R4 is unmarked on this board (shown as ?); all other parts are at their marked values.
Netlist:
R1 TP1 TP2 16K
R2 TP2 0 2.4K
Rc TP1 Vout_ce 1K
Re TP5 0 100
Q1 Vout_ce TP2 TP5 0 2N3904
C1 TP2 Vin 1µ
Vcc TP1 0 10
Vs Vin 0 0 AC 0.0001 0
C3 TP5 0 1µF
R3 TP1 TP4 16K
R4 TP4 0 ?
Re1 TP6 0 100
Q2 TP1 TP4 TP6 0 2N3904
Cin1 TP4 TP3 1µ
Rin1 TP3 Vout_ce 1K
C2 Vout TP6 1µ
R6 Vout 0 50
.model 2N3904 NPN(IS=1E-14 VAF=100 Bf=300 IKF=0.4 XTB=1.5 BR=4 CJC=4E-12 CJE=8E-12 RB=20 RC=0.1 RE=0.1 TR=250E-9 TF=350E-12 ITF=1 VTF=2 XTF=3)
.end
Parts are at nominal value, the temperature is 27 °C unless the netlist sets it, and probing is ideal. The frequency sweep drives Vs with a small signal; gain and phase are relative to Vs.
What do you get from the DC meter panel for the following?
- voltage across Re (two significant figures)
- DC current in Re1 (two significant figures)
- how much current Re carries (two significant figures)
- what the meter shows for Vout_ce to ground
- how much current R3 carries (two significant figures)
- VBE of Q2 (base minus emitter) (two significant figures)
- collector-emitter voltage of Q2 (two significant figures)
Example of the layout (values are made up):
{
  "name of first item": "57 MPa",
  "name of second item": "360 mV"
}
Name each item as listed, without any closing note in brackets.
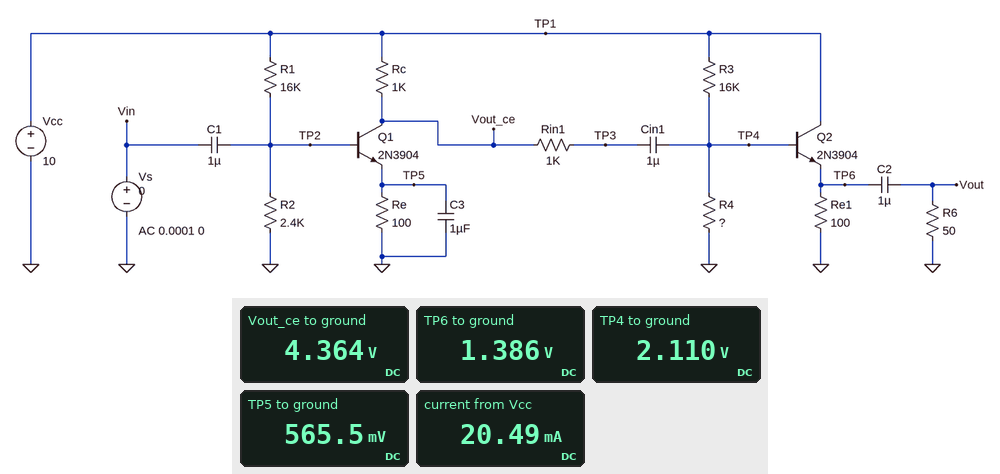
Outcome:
{
  "voltage across Re": "570 mV",
  "DC current in Re1": "14 mA",
  "how much current Re carries": "5.7 mA",
  "what the meter shows for Vout_ce to ground": "4.364 V",
  "how much current R3 carries": "490 µA",
  "VBE of Q2 (base minus emitter)": "720 mV",
  "collector-emitter voltage of Q2": "8.6 V"
}
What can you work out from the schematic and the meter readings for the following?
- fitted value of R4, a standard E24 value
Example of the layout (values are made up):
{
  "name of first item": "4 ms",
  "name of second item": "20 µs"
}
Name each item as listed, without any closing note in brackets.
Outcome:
{
  "fitted value of R4, a standard E24 value": "4.7 kΩ"
}
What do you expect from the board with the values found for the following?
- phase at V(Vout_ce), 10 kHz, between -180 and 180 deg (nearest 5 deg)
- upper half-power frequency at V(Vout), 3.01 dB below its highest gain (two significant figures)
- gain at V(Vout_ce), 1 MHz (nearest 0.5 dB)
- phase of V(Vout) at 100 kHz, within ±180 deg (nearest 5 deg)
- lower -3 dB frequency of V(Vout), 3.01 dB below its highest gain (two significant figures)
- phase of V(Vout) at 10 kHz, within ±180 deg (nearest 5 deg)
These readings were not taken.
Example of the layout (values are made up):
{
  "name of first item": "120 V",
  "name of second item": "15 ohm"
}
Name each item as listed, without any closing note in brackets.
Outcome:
{
  "phase at V(Vout_ce), 10 kHz, between -180 and 180 deg": "-115 deg",
  "upper half-power frequency at V(Vout), 3.01 dB below its highest gain": "7.7 MHz",
  "gain at V(Vout_ce), 1 MHz": "44.0 dB",
  "phase of V(Vout) at 100 kHz, within ±180 deg": "-160 deg",
  "lower -3 dB frequency of V(Vout), 3.01 dB below its highest gain": "33 kHz",
  "phase of V(Vout) at 10 kHz, within ±180 deg": "-100 deg"
}
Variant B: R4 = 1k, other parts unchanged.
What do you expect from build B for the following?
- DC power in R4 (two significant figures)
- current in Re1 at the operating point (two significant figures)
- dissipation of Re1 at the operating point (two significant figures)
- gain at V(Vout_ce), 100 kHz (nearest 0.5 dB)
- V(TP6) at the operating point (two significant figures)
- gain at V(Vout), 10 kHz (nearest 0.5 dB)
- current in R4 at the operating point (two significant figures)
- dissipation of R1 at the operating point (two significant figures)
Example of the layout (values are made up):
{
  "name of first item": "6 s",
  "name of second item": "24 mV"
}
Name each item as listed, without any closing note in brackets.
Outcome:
{
  "DC power in R4": "350 µW",
  "current in Re1 at the operating point": "64 µA",
  "dissipation of Re1 at the operating point": "410 nW",
  "gain at V(Vout_ce), 100 kHz": "42.0 dB",
  "V(TP6) at the operating point": "6.4 mV",
  "gain at V(Vout), 10 kHz": "3.0 dB",
  "current in R4 at the operating point": "590 µA",
  "dissipation of R1 at the operating point": "4.8 mW"
}
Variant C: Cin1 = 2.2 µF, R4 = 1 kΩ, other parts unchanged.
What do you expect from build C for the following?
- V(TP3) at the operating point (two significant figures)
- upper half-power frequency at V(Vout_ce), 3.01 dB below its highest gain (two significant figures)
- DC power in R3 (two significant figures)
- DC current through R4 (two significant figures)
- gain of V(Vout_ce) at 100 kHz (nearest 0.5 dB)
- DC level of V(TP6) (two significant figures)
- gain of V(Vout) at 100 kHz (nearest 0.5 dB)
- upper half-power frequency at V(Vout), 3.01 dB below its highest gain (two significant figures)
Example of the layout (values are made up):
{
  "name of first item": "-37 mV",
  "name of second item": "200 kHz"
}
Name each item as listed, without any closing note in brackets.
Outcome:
{
  "V(TP3) at the operating point": "4.4 V",
  "upper half-power frequency at V(Vout_ce), 3.01 dB below its highest gain": "14 MHz",
  "DC power in R3": "5.5 mW",
  "DC current through R4": "590 µA",
  "gain of V(Vout_ce) at 100 kHz": "42.0 dB",
  "DC level of V(TP6)": "6.4 mV",
  "gain of V(Vout) at 100 kHz": "13.5 dB",
  "upper half-power frequency at V(Vout), 3.01 dB below its highest gain": "12 MHz"
}
